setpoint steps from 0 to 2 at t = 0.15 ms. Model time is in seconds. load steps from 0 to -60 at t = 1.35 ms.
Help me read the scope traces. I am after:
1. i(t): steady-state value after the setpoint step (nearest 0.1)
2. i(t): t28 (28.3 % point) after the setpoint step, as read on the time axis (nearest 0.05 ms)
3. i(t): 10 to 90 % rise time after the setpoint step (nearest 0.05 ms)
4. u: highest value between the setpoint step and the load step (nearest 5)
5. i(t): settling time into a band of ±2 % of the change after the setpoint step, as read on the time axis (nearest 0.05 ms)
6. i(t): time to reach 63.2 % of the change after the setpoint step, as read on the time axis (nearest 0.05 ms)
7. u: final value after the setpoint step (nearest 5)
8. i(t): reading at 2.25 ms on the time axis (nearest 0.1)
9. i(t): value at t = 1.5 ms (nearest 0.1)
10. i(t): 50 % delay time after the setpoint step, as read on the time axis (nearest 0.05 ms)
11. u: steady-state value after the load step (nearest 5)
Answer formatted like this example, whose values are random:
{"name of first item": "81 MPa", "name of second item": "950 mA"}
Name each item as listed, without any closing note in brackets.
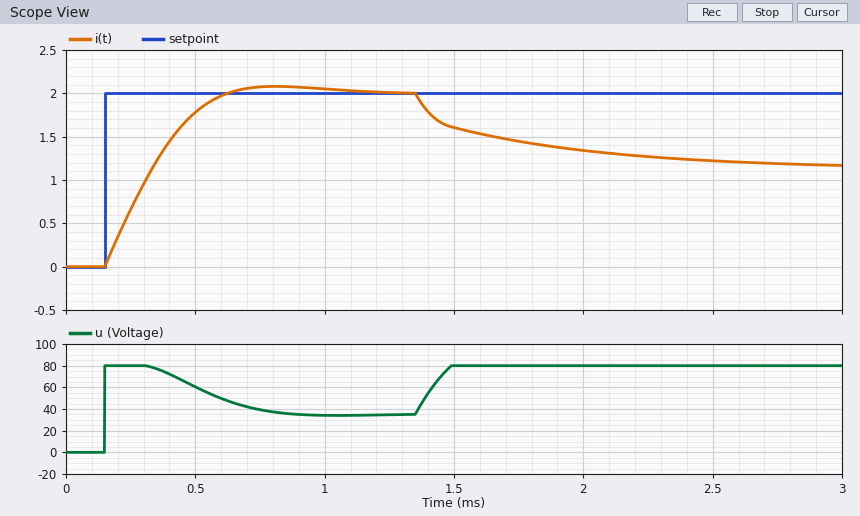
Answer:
{"i(t): steady-state value after the setpoint step": "2.0", "i(t): t28 (28.3 % point) after the setpoint step, as read on the time axis": "0.25 ms", "i(t): 10 to 90 % rise time after the setpoint step": "0.35 ms", "u: highest value between the setpoint step and the load step": "80", "i(t): settling time into a band of ±2 % of the change after the setpoint step, as read on the time axis": "1.05 ms", "i(t): time to reach 63.2 % of the change after the setpoint step, as read on the time axis": "0.35 ms", "u: final value after the setpoint step": "35", "i(t): reading at 2.25 ms on the time axis": "1.3", "i(t): value at t = 1.5 ms": "1.6", "i(t): 50 % delay time after the setpoint step, as read on the time axis": "0.30 ms", "u: steady-state value after the load step": "80"}
